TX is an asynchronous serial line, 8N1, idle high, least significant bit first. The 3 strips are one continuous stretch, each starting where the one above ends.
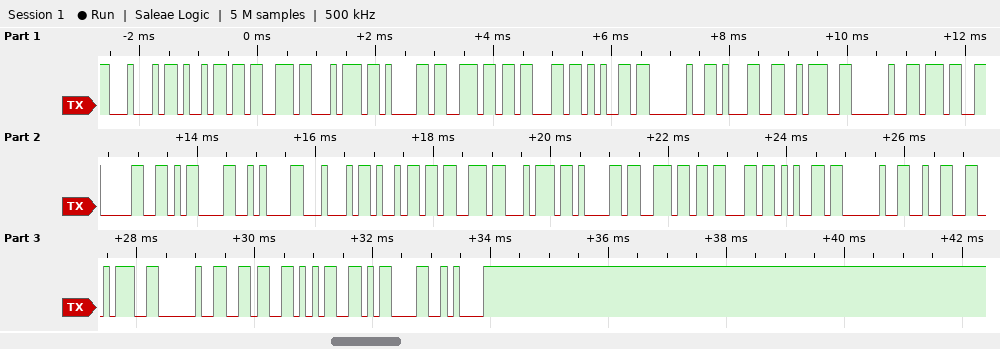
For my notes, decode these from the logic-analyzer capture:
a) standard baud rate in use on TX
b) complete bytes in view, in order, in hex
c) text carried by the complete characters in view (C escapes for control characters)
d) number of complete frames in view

9600 baud
44 69 73 74 61 6E 63 65 20 31 3A 20 37 30 0D 0A 44 69 73 74 61 6E 63 65 20 32 3A 20 36 35 0D 0A
"Distance 1: 70\r\nDistance 2: 65\r\n"
32
